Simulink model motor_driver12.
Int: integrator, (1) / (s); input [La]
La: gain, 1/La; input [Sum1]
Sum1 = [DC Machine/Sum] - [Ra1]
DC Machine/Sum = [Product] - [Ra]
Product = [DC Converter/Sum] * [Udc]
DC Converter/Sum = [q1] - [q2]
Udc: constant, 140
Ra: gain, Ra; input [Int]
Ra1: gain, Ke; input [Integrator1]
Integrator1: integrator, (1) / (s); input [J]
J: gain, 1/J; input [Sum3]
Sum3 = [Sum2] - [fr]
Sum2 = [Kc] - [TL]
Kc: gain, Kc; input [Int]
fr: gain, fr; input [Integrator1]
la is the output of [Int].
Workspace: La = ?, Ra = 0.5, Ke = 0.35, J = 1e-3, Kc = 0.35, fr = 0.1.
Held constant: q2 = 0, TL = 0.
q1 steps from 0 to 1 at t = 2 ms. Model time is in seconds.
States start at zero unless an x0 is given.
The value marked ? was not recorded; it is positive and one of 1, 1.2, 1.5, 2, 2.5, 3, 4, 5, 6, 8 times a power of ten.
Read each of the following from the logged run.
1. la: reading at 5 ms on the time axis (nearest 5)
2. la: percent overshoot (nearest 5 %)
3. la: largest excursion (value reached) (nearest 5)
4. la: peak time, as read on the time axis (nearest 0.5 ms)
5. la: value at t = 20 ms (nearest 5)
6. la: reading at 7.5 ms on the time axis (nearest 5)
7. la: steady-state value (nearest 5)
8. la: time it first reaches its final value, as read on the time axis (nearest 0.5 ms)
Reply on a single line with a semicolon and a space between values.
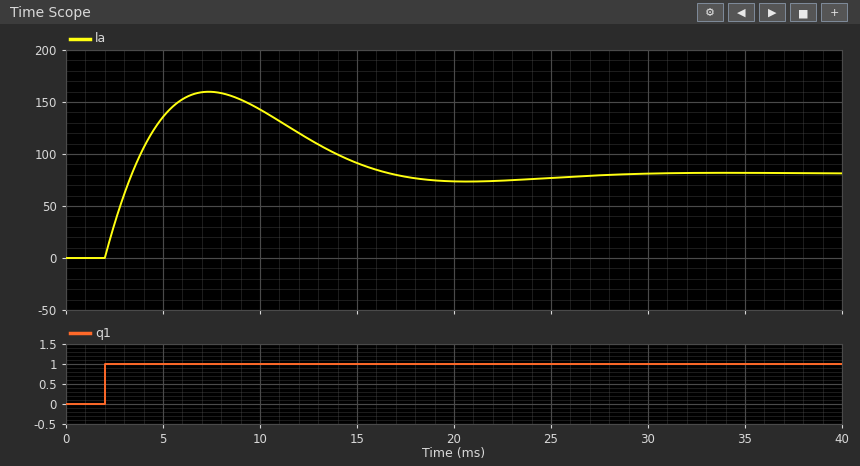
135; 95 %; 160; 7.5 ms; 75; 160; 80; 3.5 ms
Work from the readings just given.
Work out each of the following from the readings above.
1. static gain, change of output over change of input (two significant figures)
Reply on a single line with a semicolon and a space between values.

80
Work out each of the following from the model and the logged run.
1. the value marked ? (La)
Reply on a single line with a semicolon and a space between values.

0.002
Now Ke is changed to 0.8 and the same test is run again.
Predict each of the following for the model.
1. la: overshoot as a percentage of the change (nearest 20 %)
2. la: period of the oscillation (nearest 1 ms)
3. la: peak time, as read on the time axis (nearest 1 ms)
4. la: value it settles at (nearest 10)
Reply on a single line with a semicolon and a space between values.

200 %; 17 ms; 6 ms; 40
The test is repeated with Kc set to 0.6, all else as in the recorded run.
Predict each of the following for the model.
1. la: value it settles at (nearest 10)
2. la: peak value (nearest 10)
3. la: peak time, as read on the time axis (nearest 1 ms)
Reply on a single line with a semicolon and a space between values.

50; 140; 6 ms
